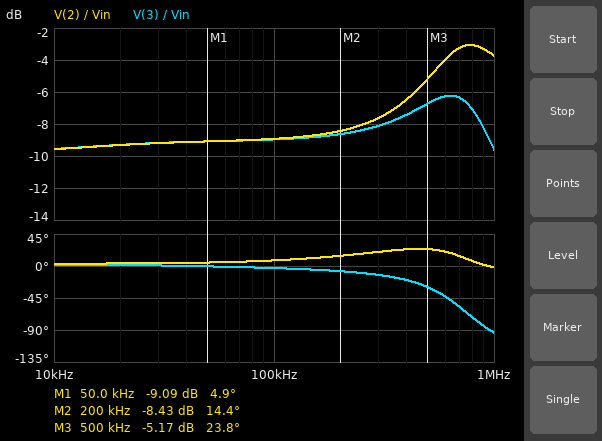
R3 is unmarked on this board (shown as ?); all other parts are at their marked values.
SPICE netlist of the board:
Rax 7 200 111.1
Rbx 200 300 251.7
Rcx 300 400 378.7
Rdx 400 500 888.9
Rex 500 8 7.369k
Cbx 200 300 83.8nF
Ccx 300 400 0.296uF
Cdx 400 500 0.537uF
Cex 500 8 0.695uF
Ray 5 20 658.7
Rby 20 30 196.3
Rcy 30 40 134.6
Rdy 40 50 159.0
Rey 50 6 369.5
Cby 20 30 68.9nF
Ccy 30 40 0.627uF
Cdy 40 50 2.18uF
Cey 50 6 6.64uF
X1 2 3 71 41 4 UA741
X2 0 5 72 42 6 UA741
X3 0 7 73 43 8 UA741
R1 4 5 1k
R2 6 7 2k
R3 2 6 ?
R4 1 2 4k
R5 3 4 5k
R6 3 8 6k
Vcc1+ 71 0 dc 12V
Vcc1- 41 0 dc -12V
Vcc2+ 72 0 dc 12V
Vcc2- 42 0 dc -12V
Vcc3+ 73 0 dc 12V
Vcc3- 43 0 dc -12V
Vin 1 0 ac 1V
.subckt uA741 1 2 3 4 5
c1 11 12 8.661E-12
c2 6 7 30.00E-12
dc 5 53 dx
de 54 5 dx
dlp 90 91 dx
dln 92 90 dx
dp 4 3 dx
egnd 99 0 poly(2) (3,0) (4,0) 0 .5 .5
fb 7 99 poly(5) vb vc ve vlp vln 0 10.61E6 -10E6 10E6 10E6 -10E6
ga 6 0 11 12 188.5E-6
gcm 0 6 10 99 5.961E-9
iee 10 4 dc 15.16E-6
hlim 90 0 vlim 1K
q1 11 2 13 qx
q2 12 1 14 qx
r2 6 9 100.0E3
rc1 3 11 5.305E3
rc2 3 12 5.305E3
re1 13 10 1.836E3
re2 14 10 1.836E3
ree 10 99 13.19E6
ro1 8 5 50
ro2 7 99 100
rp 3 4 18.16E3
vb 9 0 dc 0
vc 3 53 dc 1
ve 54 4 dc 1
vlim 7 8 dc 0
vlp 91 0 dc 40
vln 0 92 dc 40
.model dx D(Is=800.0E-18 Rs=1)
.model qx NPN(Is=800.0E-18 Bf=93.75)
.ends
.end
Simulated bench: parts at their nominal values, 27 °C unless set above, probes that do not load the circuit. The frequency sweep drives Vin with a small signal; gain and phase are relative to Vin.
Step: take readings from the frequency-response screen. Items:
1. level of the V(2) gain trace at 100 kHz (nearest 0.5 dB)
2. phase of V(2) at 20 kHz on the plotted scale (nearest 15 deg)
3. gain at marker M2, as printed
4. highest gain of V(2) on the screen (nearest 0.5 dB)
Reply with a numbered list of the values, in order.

1. -9.0 dB
2. 0 deg
3. -8.43 dB
4. -3.0 dB
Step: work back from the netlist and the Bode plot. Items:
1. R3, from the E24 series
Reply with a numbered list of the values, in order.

1. 4.7 kΩ
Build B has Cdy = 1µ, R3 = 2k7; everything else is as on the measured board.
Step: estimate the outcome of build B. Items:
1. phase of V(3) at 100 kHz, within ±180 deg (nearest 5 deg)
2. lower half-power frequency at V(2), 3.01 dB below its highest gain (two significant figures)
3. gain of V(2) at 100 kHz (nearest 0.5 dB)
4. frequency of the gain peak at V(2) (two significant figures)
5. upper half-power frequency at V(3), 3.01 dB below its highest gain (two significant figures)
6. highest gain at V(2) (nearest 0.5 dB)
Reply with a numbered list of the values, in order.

1. 0 deg
2. 510 kHz
3. -12.5 dB
4. 790 kHz
5. 980 kHz
6. -5.0 dB
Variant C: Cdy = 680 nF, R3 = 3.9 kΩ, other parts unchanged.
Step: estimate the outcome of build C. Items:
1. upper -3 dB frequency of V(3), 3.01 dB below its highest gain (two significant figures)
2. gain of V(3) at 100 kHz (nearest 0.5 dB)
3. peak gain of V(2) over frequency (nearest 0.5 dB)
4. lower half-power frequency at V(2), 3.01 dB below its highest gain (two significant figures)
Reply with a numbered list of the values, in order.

1. 980 kHz
2. -10.0 dB
3. -3.5 dB
4. 460 kHz
